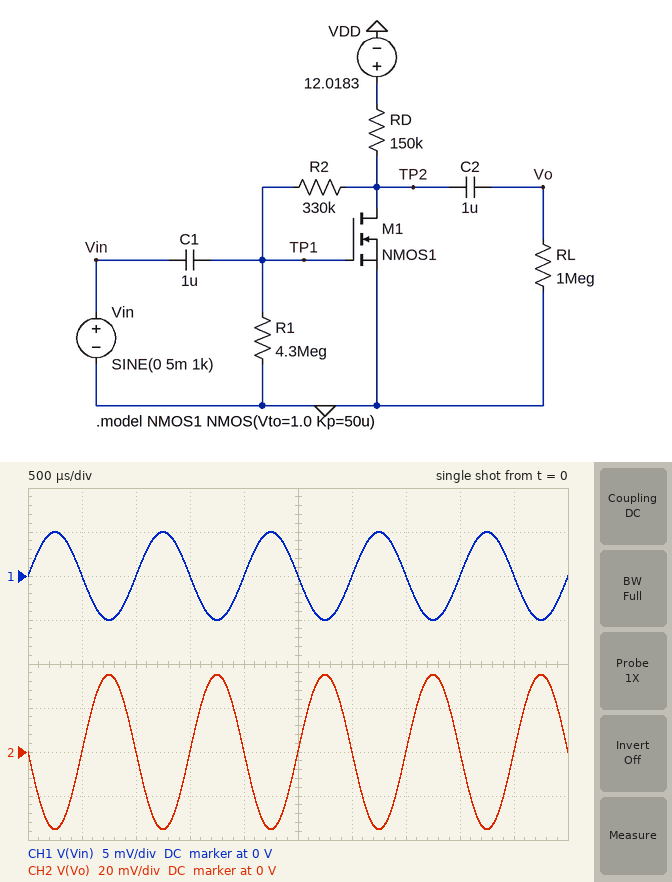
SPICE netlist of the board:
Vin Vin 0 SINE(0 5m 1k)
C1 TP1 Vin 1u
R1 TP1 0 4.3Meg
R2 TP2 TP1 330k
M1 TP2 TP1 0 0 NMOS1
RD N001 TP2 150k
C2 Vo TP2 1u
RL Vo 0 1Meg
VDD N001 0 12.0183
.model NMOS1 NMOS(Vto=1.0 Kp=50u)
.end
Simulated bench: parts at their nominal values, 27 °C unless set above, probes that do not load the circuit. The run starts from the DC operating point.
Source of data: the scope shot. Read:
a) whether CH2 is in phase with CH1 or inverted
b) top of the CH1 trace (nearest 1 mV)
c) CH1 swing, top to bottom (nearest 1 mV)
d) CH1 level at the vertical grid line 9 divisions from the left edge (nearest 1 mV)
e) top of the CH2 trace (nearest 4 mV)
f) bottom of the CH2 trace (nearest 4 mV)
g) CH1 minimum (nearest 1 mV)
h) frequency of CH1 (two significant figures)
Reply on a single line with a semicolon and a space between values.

inverted; 5 mV; 10 mV; 0 V; 36 mV; -36 mV; -5 mV; 1.0 kHz
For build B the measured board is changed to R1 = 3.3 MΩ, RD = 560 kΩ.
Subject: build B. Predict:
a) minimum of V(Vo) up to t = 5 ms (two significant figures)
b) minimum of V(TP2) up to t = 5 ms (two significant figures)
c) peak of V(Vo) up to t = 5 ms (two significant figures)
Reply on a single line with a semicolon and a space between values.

-33 mV; 2.0 V; 33 mV
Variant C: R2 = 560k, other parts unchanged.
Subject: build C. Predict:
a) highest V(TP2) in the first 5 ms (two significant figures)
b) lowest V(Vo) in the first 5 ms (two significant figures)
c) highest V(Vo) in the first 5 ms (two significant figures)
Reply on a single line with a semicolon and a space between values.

2.9 V; -40 mV; 40 mV
